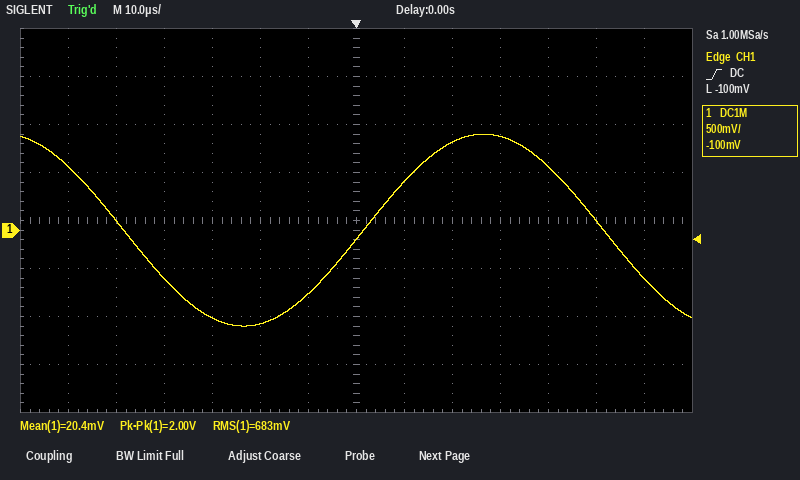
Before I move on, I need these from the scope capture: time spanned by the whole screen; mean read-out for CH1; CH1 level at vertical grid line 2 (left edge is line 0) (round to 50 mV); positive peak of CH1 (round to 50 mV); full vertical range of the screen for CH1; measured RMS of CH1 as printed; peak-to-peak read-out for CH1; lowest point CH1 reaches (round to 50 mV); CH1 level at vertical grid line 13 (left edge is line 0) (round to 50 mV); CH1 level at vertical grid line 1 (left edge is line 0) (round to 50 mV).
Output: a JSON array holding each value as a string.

["140 µs", "20.4 mV", "100 mV", "1.00 V", "4 V", "683 mV", "2.00 V", "-1.00 V", "-500 mV", "650 mV"]
